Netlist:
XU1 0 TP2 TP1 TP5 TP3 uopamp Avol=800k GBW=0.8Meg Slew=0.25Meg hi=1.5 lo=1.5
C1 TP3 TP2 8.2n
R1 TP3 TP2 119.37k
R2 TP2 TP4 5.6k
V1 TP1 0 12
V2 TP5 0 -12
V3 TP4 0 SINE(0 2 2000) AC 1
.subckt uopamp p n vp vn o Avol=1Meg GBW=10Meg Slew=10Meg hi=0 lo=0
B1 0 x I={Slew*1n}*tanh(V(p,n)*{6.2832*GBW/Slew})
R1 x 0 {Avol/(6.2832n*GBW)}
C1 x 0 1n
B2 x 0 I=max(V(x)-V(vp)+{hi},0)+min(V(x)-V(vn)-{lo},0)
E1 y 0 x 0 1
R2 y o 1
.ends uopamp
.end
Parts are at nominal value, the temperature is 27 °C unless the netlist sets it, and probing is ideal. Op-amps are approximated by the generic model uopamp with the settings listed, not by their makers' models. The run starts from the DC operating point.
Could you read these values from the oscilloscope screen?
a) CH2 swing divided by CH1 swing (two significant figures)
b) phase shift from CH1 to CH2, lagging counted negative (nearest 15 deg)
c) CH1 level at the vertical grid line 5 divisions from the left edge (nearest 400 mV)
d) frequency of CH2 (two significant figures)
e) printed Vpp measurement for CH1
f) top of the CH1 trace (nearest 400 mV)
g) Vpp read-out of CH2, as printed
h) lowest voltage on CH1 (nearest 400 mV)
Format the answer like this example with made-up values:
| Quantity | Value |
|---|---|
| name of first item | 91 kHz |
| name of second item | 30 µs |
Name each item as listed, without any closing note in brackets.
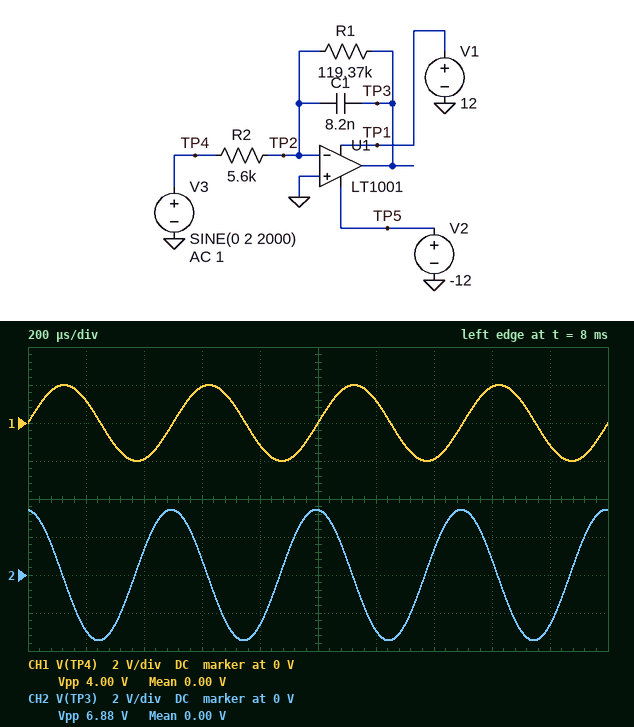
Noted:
| Quantity | Value |
|---|---|
| CH2 swing divided by CH1 swing | 1.7 |
| phase shift from CH1 to CH2, lagging counted negative | 90 deg |
| CH1 level at the vertical grid line 5 divisions from the left edge | 0 V |
| frequency of CH2 | 2.0 kHz |
| printed Vpp measurement for CH1 | 4.00 V |
| top of the CH1 trace | 2.0 V |
| Vpp read-out of CH2, as printed | 6.88 V |
| lowest voltage on CH1 | -2.0 V |
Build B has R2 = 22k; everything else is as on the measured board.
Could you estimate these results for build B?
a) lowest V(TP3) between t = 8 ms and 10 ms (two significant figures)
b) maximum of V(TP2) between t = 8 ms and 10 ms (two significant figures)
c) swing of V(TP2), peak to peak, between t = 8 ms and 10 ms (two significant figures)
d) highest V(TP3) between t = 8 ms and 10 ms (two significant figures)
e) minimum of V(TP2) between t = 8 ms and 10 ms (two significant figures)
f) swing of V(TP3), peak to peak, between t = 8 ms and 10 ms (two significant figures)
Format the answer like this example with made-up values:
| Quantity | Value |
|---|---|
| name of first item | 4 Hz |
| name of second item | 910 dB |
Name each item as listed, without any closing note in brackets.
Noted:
| Quantity | Value |
|---|---|
| lowest V(TP3) between t = 8 ms and 10 ms | -880 mV |
| maximum of V(TP2) between t = 8 ms and 10 ms | 2.2 mV |
| swing of V(TP2), peak to peak, between t = 8 ms and 10 ms | 4.4 mV |
| highest V(TP3) between t = 8 ms and 10 ms | 880 mV |
| minimum of V(TP2) between t = 8 ms and 10 ms | -2.2 mV |
| swing of V(TP3), peak to peak, between t = 8 ms and 10 ms | 1.8 V |
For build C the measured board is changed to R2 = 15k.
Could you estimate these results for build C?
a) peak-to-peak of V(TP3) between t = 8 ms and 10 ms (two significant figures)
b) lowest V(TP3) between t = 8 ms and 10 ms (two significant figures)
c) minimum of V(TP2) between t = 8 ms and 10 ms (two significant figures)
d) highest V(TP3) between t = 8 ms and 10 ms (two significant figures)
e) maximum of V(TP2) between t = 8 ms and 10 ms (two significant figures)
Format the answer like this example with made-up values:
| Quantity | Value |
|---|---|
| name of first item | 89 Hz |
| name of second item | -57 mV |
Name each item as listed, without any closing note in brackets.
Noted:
| Quantity | Value |
|---|---|
| peak-to-peak of V(TP3) between t = 8 ms and 10 ms | 2.6 V |
| lowest V(TP3) between t = 8 ms and 10 ms | -1.3 V |
| minimum of V(TP2) between t = 8 ms and 10 ms | -3.2 mV |
| highest V(TP3) between t = 8 ms and 10 ms | 1.3 V |
| maximum of V(TP2) between t = 8 ms and 10 ms | 3.2 mV |
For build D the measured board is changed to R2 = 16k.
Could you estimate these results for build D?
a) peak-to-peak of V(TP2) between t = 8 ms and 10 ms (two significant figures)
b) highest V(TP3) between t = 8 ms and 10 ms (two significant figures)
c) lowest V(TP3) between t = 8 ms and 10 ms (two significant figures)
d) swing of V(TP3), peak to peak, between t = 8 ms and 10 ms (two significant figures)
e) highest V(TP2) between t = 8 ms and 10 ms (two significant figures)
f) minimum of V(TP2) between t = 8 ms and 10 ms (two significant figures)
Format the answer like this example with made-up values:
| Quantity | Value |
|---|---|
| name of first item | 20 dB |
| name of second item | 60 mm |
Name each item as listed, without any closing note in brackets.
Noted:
| Quantity | Value |
|---|---|
| peak-to-peak of V(TP2) between t = 8 ms and 10 ms | 6.0 mV |
| highest V(TP3) between t = 8 ms and 10 ms | 1.2 V |
| lowest V(TP3) between t = 8 ms and 10 ms | -1.2 V |
| swing of V(TP3), peak to peak, between t = 8 ms and 10 ms | 2.4 V |
| highest V(TP2) between t = 8 ms and 10 ms | 3.0 mV |
| minimum of V(TP2) between t = 8 ms and 10 ms | -3.0 mV |
